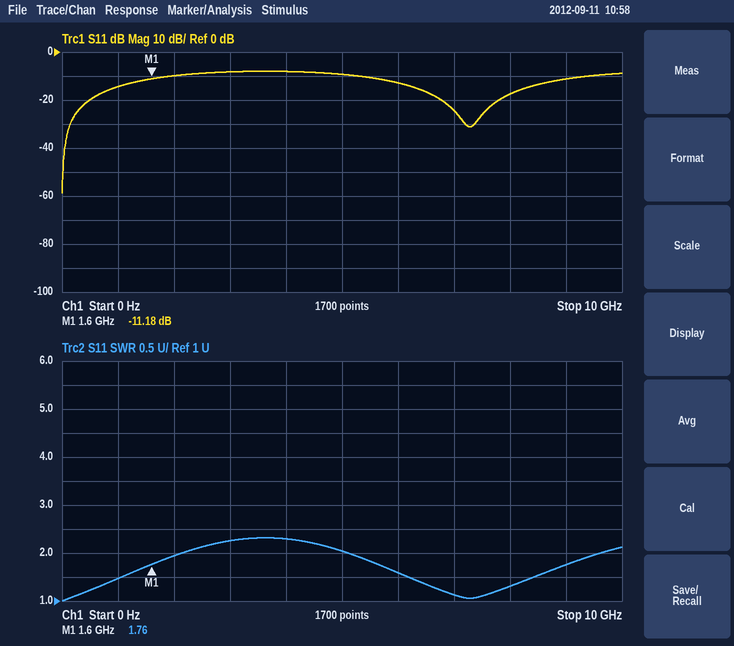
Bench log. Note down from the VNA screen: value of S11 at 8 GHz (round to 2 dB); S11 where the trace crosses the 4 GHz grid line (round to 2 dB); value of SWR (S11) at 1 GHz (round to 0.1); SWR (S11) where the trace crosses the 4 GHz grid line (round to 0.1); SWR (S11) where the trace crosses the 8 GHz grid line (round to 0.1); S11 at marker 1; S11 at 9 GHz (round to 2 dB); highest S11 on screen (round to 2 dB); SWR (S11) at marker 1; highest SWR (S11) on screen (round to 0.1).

-18 dB
-8 dB
1.5
2.3
1.3
-11.18 dB
-12 dB
-8 dB
1.76
2.3
